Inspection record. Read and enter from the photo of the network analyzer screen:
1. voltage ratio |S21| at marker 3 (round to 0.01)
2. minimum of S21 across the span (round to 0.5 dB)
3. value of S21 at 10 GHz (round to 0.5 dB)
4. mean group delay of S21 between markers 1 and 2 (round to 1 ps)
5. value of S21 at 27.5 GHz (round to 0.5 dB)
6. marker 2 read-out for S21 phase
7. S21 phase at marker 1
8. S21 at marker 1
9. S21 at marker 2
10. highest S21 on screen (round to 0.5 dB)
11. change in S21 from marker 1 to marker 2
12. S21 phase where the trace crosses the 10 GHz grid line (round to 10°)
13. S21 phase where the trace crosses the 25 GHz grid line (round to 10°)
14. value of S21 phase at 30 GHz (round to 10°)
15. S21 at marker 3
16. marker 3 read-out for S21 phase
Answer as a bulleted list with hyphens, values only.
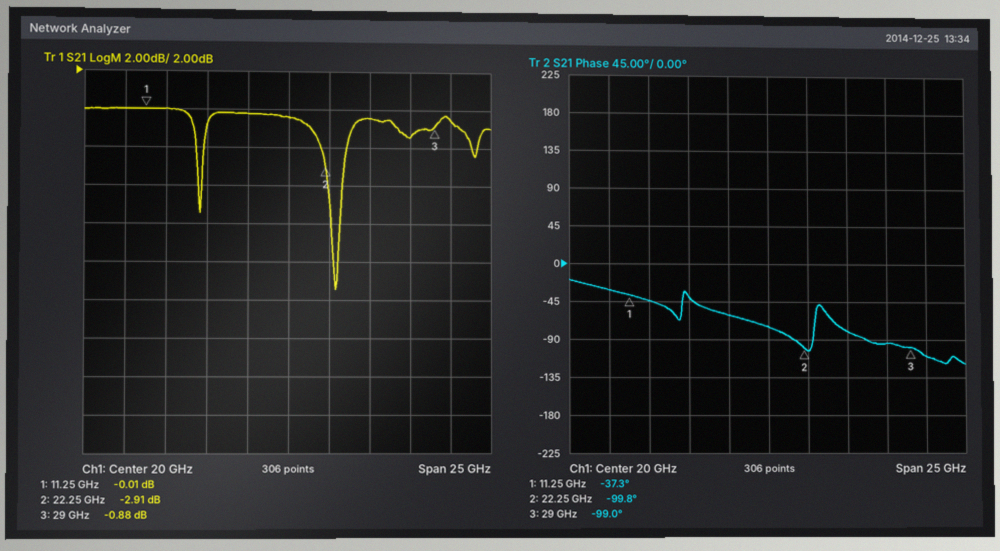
- 0.90
- -9.5 dB
- 0.0 dB
- 16 ps
- -1.5 dB
- -99.8°
- -37.3°
- -0.01 dB
- -2.91 dB
- 0.0 dB
- -2.90 dB
- -30°
- -80°
- -110°
- -0.88 dB
- -99.0°
